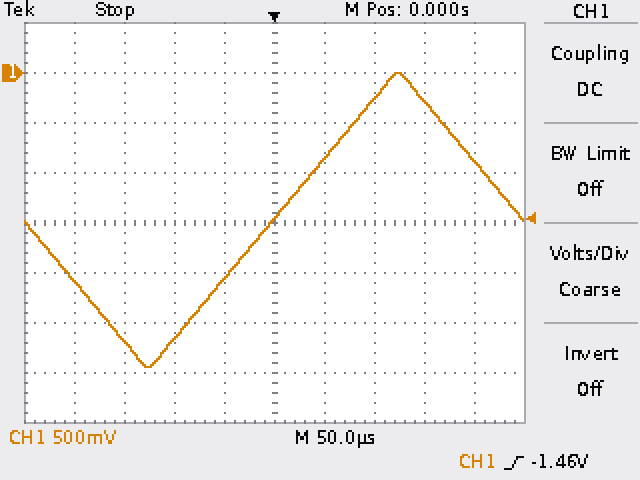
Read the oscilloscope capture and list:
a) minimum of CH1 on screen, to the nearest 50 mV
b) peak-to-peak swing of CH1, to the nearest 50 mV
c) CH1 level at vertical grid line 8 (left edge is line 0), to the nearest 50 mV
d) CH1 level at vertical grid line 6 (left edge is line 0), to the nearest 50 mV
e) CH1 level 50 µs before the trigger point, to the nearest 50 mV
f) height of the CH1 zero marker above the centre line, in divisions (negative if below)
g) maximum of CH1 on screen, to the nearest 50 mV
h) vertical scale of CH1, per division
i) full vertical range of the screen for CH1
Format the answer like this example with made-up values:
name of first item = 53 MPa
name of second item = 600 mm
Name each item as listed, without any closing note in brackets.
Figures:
minimum of CH1 on screen, to the nearest 50 mV = -2.95 V
peak-to-peak swing of CH1, to the nearest 50 mV = 2.95 V
CH1 level at vertical grid line 8 (left edge is line 0), to the nearest 50 mV = -300 mV
CH1 level at vertical grid line 6 (left edge is line 0), to the nearest 50 mV = -850 mV
CH1 level 50 µs before the trigger point, to the nearest 50 mV = -2.05 V
height of the CH1 zero marker above the centre line, in divisions = +3.0 div
maximum of CH1 on screen, to the nearest 50 mV = 0 mV
vertical scale of CH1, per division = 500 mV
full vertical range of the screen for CH1 = 4 V
